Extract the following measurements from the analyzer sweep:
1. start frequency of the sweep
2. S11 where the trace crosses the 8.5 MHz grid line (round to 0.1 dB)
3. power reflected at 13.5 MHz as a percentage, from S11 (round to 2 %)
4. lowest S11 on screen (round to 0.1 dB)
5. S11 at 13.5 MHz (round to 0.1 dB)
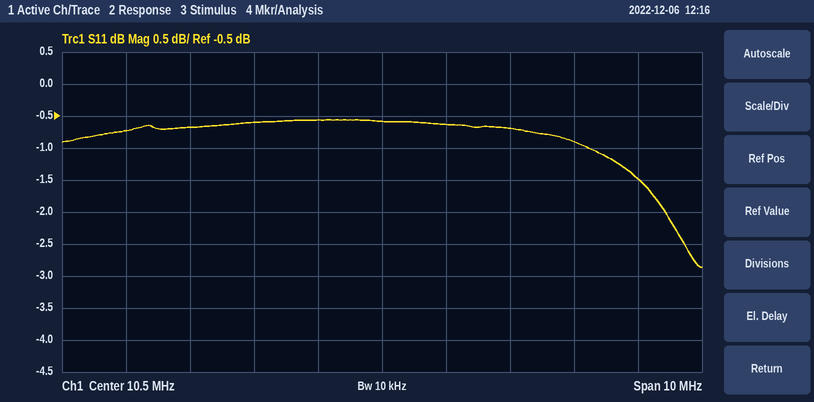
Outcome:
5.5 MHz
-0.6 dB
82 %
-2.9 dB
-0.9 dB
